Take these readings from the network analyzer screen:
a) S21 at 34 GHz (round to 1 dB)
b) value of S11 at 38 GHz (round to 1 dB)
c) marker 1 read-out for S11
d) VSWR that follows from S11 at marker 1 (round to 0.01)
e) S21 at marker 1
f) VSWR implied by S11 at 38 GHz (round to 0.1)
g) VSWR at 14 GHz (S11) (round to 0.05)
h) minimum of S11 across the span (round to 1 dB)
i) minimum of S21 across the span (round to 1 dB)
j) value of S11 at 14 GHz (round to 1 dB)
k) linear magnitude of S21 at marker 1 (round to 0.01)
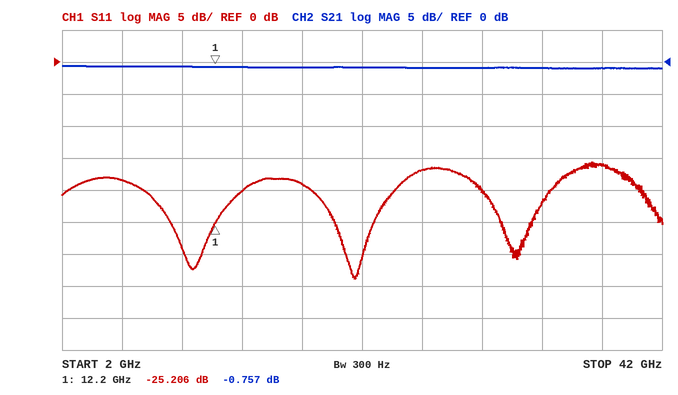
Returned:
-1 dB
-16 dB
-25.206 dB
1.12
-0.757 dB
1.4
1.20
-34 dB
-1 dB
-20 dB
0.92
